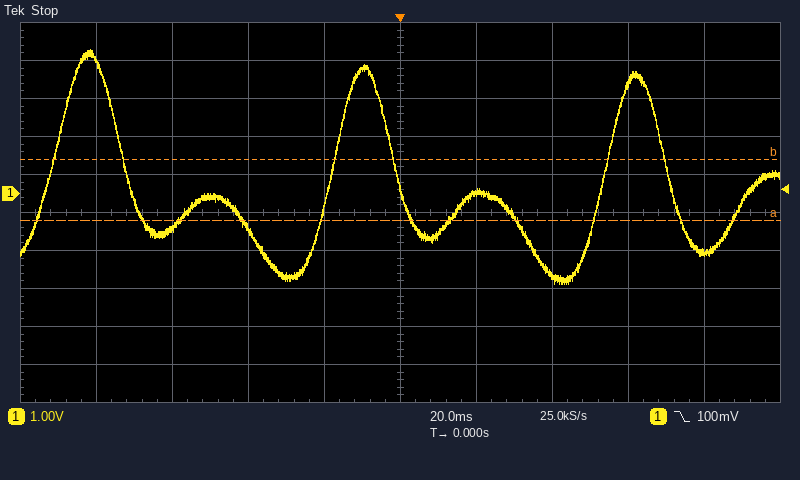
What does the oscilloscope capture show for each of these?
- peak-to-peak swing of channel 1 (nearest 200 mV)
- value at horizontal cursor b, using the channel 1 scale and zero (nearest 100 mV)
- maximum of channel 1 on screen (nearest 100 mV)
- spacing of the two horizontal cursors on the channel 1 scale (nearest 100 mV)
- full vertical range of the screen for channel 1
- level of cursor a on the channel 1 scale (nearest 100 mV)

6.2 V
900 mV
3.8 V
1.6 V
10 V
-700 mV
